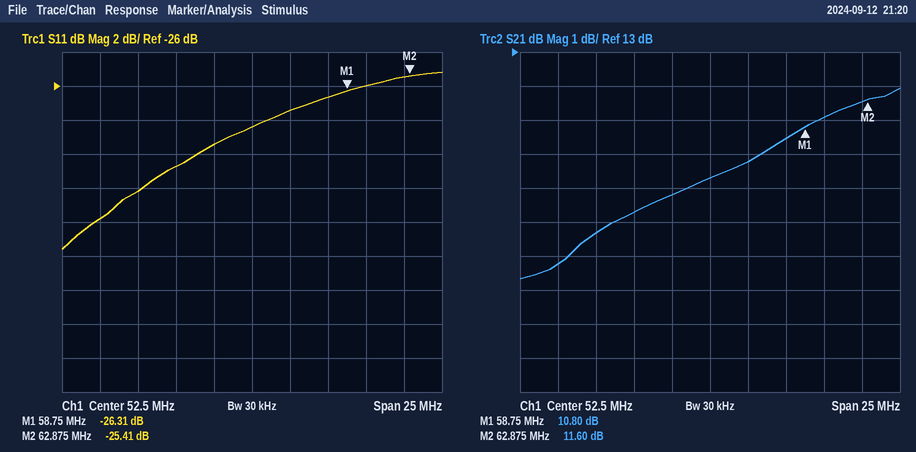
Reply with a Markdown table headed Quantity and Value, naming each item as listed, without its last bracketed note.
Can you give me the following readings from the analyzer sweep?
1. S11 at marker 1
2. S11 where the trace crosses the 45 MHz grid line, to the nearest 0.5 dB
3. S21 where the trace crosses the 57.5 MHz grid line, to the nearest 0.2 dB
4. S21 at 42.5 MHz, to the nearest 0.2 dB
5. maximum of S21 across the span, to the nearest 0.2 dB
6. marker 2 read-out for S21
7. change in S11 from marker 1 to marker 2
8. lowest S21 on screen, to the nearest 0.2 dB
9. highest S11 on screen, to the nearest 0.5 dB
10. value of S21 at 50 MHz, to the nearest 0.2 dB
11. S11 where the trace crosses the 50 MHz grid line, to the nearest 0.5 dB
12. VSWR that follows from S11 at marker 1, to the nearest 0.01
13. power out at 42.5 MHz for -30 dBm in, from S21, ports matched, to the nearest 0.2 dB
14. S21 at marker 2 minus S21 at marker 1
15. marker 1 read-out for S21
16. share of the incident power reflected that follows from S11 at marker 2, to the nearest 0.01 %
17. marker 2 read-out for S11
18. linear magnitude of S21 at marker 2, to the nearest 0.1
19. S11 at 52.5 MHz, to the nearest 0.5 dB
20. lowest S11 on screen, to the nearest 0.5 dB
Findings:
| Quantity | Value |
|---|---|
| S11 at marker 1 | -26.31 dB |
| S11 where the trace crosses the 45 MHz grid line, to the nearest 0.5 dB | -32.0 dB |
| S21 where the trace crosses the 57.5 MHz grid line, to the nearest 0.2 dB | 10.4 dB |
| S21 at 42.5 MHz, to the nearest 0.2 dB | 6.8 dB |
| maximum of S21 across the span, to the nearest 0.2 dB | 12.0 dB |
| marker 2 read-out for S21 | 11.60 dB |
| change in S11 from marker 1 to marker 2 | 0.90 dB |
| lowest S21 on screen, to the nearest 0.2 dB | 6.4 dB |
| highest S11 on screen, to the nearest 0.5 dB | -25.0 dB |
| value of S21 at 50 MHz, to the nearest 0.2 dB | 8.8 dB |
| S11 where the trace crosses the 50 MHz grid line, to the nearest 0.5 dB | -29.5 dB |
| VSWR that follows from S11 at marker 1, to the nearest 0.01 | 1.10 |
| power out at 42.5 MHz for -30 dBm in, from S21, ports matched, to the nearest 0.2 dB | -23.2 dBm |
| S21 at marker 2 minus S21 at marker 1 | 0.80 dB |
| marker 1 read-out for S21 | 10.80 dB |
| share of the incident power reflected that follows from S11 at marker 2, to the nearest 0.01 % | 0.29 % |
| marker 2 read-out for S11 | -25.41 dB |
| linear magnitude of S21 at marker 2, to the nearest 0.1 | 3.8 |
| S11 at 52.5 MHz, to the nearest 0.5 dB | -28.5 dB |
| lowest S11 on screen, to the nearest 0.5 dB | -35.5 dB |
